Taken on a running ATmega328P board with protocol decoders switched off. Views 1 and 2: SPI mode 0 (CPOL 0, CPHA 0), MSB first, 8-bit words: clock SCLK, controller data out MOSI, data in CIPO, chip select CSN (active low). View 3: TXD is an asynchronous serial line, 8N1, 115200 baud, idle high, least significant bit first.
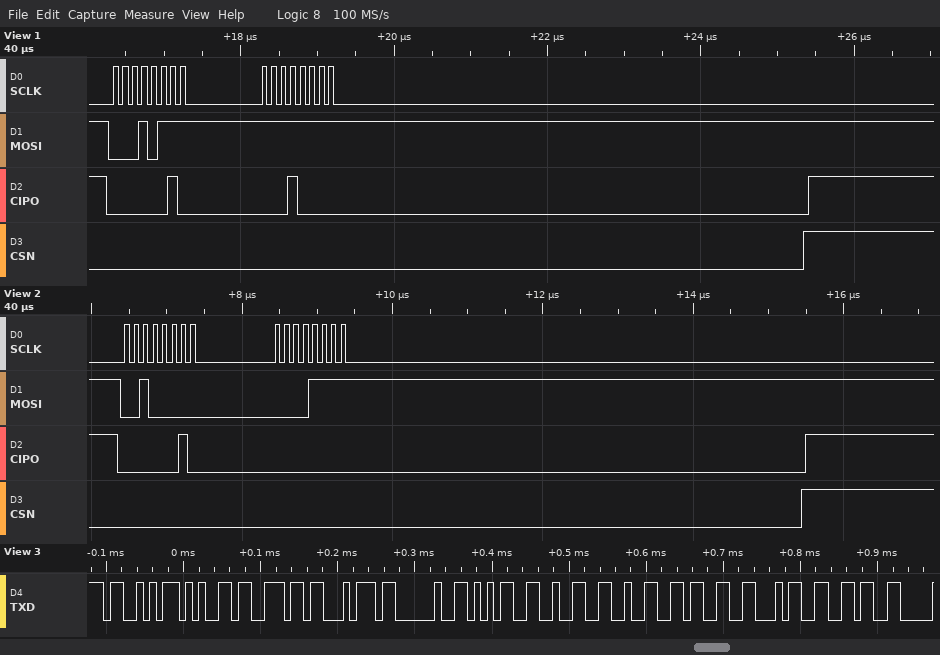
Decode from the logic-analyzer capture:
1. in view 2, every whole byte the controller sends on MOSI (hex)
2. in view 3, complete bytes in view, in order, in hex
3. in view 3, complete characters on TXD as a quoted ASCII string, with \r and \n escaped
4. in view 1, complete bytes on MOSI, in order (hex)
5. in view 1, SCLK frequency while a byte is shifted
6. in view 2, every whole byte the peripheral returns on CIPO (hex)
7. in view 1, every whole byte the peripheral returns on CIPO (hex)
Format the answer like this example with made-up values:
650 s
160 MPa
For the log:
20 0F
0x53 0x65 0x6E 0x74 0x20 0x35 0x32 0x32 0x33 0x34 0x36
"Sent 522346"
17 FF
8 MHz
02 00
02 10
